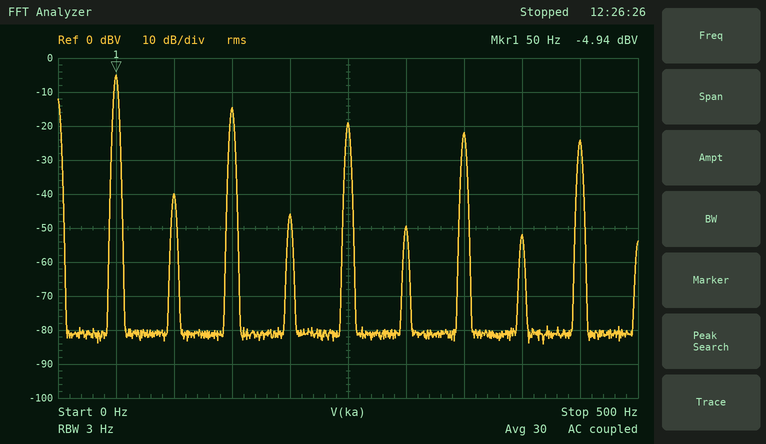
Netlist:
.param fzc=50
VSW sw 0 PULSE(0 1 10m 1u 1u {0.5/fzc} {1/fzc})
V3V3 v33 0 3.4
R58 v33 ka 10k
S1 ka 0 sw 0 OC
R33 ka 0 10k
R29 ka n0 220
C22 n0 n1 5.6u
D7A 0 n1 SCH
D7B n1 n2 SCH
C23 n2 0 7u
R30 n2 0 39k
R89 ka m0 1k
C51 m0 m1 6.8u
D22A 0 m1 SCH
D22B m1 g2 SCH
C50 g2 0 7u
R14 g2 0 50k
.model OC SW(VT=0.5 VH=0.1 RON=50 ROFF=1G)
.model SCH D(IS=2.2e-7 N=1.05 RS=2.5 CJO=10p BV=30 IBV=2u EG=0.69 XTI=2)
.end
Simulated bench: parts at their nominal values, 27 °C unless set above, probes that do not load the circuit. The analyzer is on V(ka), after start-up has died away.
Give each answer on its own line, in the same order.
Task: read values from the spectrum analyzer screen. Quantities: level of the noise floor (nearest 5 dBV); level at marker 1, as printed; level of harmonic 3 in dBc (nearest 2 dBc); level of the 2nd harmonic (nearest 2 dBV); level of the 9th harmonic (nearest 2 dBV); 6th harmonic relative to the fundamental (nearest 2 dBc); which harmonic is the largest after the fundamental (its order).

-80 dBV
-4.94 dBV
-10 dBc
-40 dBV
-24 dBV
-44 dBc
3
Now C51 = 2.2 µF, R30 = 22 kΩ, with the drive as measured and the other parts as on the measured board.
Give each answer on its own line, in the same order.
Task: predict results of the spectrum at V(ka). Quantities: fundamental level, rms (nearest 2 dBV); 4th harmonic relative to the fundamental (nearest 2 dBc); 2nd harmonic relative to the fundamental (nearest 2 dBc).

-6 dBV
-36 dBc
-30 dBc
